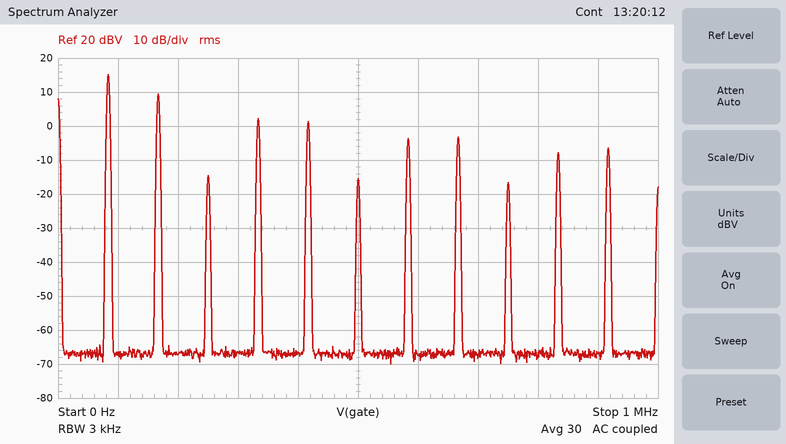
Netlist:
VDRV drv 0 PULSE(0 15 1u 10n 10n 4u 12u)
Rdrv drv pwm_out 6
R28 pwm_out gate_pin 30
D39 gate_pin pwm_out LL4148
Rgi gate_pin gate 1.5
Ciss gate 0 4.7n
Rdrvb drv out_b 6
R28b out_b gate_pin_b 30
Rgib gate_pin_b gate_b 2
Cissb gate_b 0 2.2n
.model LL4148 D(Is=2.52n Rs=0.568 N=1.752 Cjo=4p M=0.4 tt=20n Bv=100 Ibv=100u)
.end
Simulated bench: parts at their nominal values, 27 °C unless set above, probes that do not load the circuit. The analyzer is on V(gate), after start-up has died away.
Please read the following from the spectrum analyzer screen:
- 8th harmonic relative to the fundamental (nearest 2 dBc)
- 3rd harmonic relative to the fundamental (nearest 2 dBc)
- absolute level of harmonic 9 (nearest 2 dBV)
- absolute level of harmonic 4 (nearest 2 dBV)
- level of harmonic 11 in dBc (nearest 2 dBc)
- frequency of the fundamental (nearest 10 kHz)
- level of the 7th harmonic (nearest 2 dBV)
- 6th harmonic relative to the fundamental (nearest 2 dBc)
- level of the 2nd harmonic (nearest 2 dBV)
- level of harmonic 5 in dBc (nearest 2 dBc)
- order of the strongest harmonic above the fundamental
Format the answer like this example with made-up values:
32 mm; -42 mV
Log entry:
-18 dBc; -30 dBc; -16 dBV; 2 dBV; -22 dBc; 80 kHz; -4 dBV; -30 dBc; 10 dBV; -14 dBc; 2
